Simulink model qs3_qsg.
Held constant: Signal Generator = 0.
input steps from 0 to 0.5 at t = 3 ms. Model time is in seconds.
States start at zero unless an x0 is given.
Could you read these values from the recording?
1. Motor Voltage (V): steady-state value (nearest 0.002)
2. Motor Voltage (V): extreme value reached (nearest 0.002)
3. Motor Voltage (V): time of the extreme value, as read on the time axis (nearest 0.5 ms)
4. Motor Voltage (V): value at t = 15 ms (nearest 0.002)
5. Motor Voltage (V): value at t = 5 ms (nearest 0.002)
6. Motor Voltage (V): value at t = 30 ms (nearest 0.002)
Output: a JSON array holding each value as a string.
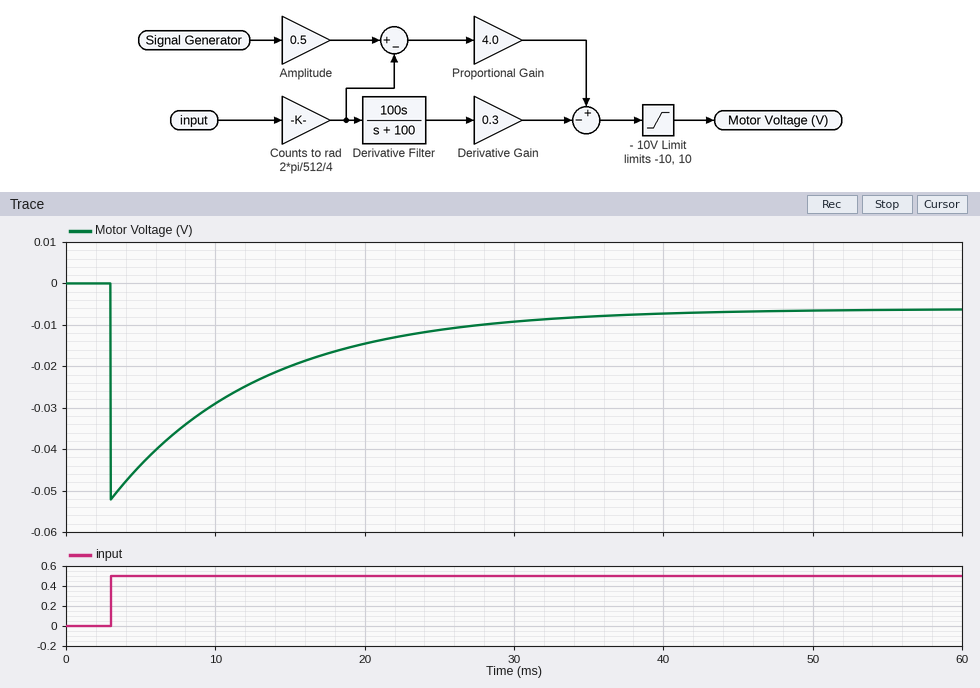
["-0.006", "-0.052", "3.0 ms", "-0.020", "-0.044", "-0.010"]
